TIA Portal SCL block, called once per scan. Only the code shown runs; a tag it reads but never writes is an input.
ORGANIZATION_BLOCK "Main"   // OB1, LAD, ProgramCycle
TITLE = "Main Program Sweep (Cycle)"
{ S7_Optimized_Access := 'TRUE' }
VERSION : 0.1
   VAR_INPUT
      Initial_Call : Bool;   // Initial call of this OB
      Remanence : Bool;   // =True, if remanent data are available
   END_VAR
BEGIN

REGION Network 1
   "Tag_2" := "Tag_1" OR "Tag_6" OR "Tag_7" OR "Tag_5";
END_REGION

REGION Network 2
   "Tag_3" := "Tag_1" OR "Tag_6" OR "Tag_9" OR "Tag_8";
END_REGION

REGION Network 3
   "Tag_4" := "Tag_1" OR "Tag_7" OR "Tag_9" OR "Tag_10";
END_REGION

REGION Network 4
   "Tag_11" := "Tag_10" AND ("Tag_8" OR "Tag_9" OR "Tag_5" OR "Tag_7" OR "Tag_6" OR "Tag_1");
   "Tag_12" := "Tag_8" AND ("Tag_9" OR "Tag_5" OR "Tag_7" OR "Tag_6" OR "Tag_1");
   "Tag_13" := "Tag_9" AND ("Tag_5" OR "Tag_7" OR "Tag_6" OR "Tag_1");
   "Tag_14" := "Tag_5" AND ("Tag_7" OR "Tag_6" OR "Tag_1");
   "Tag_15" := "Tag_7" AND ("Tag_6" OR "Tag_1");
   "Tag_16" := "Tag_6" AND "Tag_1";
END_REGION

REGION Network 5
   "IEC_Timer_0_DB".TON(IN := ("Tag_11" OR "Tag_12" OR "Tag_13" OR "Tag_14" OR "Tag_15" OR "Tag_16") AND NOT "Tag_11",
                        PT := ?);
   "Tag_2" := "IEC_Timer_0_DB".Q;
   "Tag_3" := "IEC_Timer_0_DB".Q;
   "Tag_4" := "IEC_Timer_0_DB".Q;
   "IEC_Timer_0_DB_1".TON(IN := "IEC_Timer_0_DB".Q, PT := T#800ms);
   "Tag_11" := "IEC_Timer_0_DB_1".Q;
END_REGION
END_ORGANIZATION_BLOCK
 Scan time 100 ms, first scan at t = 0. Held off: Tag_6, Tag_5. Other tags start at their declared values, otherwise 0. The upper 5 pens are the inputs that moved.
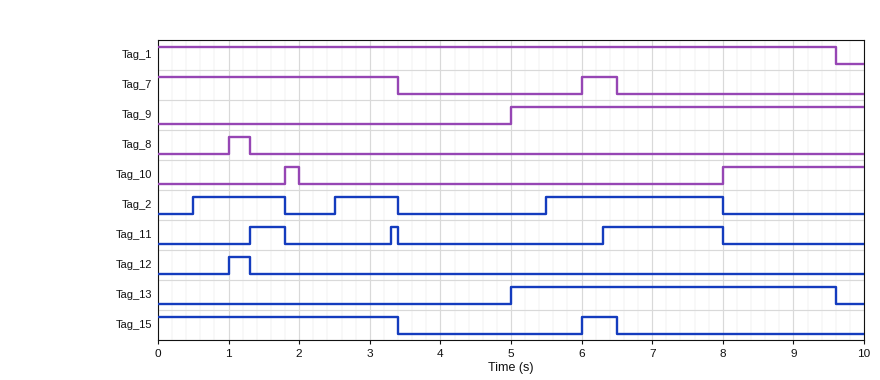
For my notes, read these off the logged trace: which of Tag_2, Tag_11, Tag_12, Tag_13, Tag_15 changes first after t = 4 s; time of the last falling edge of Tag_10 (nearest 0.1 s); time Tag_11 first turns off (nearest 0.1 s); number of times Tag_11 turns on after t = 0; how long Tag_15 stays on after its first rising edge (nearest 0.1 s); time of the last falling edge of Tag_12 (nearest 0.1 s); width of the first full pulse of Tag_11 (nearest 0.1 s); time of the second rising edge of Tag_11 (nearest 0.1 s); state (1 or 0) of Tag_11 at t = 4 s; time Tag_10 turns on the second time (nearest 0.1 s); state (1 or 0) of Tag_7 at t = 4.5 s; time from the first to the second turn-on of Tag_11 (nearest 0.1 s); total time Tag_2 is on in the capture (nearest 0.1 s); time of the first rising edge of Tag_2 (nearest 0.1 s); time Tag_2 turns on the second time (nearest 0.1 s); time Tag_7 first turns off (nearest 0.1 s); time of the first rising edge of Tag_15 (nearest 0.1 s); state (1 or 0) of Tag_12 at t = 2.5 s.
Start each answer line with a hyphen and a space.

- Tag_13
- 2.0 s
- 1.8 s
- 3
- 0.5 s
- 1.3 s
- 0.5 s
- 3.3 s
- 0
- 8.0 s
- 0
- 2.0 s
- 4.7 s
- 0.5 s
- 2.5 s
- 3.4 s
- 6.0 s
- 0
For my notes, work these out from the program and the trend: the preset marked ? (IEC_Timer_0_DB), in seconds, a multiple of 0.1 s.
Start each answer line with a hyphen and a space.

- 0.5 s
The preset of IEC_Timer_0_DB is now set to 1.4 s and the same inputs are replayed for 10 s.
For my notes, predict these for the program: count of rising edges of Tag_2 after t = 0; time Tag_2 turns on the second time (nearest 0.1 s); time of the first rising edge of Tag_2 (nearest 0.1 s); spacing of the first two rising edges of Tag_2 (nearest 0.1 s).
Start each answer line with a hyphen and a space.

- 2
- 6.4 s
- 1.4 s
- 5.0 s
